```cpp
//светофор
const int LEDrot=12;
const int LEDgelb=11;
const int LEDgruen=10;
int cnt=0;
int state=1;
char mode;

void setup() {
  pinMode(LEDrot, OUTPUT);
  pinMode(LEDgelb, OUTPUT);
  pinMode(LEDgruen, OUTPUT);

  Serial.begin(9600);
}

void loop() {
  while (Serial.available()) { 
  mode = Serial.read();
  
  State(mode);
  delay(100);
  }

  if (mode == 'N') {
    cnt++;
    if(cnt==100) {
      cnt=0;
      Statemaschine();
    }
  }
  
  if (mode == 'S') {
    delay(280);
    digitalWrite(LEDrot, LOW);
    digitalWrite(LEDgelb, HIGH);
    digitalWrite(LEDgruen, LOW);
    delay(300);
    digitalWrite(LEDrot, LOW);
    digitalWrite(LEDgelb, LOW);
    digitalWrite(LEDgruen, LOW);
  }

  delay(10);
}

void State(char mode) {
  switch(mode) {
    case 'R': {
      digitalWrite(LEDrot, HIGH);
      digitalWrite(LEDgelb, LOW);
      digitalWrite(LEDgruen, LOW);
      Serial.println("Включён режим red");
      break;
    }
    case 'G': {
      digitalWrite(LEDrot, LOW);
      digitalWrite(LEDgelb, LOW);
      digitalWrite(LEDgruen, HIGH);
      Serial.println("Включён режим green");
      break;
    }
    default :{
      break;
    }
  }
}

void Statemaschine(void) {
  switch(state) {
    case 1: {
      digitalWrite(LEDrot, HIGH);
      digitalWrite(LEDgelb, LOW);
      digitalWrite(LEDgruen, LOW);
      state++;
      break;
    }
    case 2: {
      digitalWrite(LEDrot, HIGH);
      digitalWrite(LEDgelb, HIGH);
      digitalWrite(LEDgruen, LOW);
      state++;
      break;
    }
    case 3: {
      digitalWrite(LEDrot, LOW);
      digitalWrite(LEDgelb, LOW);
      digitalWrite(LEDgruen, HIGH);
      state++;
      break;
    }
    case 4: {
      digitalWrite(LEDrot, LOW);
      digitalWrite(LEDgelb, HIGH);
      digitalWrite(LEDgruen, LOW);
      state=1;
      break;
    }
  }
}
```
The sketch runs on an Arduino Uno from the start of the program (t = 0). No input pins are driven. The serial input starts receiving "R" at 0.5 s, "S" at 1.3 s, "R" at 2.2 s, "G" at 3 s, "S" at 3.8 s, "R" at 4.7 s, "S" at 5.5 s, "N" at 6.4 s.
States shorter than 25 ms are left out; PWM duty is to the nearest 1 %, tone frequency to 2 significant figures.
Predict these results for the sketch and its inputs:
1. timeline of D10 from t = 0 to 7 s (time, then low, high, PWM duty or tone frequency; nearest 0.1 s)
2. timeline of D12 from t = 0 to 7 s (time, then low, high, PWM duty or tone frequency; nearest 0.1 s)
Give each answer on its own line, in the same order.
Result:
0 s low; 3 s high; 4.2 s low
0 s low; 0.5 s high; 1.7 s low; 2.6 s high; 3 s low; 5.1 s high; 5.9 s low
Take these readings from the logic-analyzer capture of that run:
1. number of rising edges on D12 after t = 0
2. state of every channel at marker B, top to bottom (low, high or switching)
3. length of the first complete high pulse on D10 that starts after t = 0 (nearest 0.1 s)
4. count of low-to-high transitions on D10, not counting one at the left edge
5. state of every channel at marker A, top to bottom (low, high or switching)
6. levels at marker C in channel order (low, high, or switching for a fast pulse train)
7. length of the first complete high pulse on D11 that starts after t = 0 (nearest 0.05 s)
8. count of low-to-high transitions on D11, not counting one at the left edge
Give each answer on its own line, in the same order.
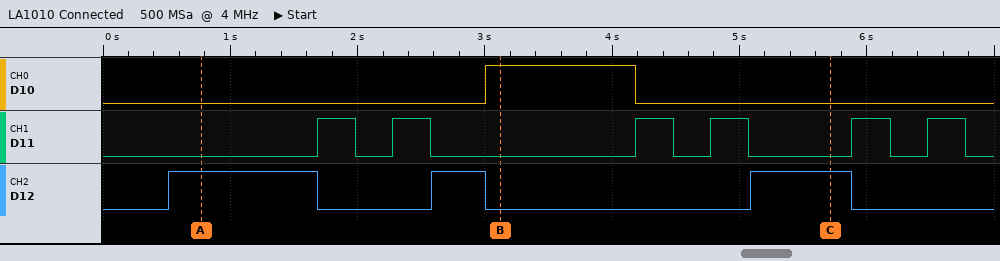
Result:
3
D10 high, D11 low, D12 low
1.2 s
1
D10 low, D11 low, D12 high
D10 low, D11 low, D12 high
0.30 s
6
